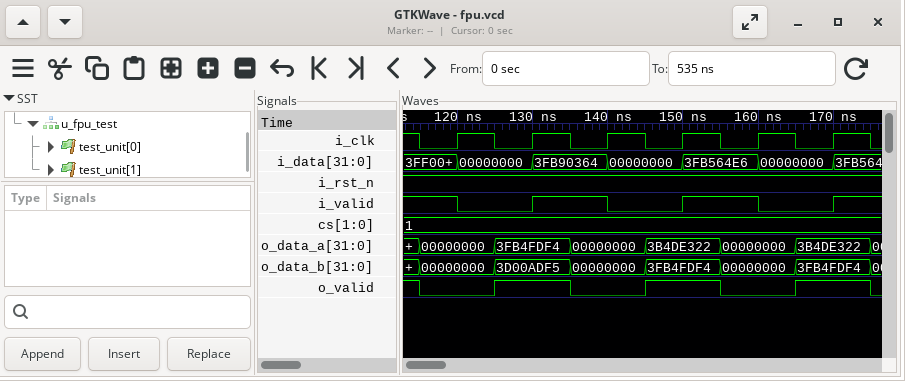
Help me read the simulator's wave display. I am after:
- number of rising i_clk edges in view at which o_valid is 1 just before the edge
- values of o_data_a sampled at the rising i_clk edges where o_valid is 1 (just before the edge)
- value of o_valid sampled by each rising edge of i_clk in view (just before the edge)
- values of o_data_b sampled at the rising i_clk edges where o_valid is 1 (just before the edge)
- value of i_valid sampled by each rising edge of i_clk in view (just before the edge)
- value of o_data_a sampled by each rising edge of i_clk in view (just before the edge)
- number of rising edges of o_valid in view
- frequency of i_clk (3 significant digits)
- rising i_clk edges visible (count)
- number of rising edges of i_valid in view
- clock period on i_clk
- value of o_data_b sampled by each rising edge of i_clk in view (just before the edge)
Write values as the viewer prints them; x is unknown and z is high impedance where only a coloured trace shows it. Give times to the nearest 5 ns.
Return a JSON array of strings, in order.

["3", "3FB4FDF4, 3B4DE322, 3B4DE322", "0 1 0 1 0 1", "3D00ADF5, 3FB4FDF4, 3FB4FDF4", "1 0 1 0 1 0", "00000000, 3FB4FDF4, 00000000, 3B4DE322, 00000000, 3B4DE322", "3", "100 MHz", "6", "3", "10 ns", "00000000, 3D00ADF5, 00000000, 3FB4FDF4, 00000000, 3FB4FDF4"]
